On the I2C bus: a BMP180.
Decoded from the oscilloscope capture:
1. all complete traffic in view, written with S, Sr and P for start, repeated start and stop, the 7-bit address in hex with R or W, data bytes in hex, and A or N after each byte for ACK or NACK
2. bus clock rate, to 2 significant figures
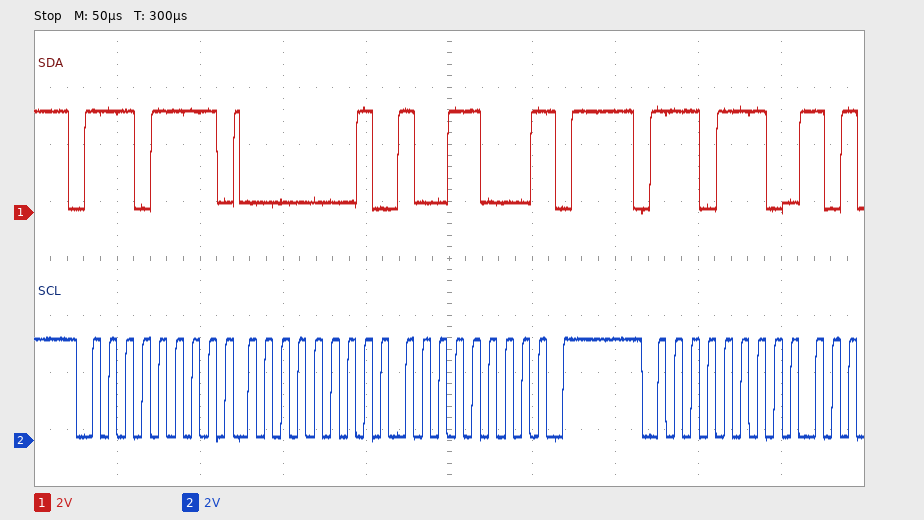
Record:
S 77R A 01 A 98 N P S 77W A
100 kHz
